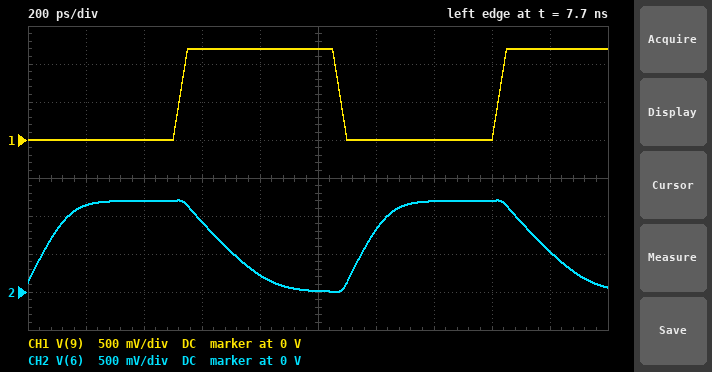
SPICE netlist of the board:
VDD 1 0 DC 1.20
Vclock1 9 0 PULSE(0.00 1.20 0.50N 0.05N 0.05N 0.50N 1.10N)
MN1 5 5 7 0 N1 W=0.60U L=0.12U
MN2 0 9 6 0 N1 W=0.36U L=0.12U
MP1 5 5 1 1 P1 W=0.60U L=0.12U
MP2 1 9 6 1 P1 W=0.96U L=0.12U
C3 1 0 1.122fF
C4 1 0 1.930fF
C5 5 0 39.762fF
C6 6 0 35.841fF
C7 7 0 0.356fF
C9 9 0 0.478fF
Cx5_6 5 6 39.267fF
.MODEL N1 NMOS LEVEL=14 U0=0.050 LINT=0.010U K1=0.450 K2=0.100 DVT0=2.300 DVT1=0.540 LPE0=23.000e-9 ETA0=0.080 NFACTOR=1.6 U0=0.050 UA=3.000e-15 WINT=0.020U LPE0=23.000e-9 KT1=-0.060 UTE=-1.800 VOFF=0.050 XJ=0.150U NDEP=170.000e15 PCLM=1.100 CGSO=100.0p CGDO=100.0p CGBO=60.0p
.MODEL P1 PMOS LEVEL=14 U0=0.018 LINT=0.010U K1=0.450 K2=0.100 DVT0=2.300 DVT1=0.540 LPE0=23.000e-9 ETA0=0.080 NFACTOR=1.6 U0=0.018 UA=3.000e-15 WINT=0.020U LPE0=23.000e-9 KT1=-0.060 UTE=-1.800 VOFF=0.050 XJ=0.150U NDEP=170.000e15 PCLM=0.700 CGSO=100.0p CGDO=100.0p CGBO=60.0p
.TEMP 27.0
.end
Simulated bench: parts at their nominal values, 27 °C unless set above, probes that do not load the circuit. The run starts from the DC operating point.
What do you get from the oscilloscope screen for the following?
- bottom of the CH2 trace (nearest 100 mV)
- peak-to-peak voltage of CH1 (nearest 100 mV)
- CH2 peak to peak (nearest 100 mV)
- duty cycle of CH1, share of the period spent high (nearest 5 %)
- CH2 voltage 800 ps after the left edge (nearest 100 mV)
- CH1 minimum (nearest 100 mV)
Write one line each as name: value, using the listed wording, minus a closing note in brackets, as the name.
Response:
bottom of the CH2 trace: 0 V
peak-to-peak voltage of CH1: 1.2 V
CH2 peak to peak: 1.2 V
duty cycle of CH1, share of the period spent high: 50 %
CH2 voltage 800 ps after the left edge: 200 mV
CH1 minimum: 0 V
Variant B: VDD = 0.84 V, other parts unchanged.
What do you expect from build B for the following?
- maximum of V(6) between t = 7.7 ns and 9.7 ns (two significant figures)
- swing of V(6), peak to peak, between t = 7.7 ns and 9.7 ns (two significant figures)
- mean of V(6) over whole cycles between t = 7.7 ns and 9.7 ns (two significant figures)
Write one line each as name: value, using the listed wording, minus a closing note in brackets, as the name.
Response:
maximum of V(6) between t = 7.7 ns and 9.7 ns: 840 mV
swing of V(6), peak to peak, between t = 7.7 ns and 9.7 ns: 850 mV
mean of V(6) over whole cycles between t = 7.7 ns and 9.7 ns: 410 mV
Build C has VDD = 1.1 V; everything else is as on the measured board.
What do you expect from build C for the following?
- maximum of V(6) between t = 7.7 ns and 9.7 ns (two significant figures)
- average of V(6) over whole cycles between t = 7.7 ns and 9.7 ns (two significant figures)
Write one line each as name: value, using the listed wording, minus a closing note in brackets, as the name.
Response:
maximum of V(6) between t = 7.7 ns and 9.7 ns: 1.1 V
average of V(6) over whole cycles between t = 7.7 ns and 9.7 ns: 600 mV
